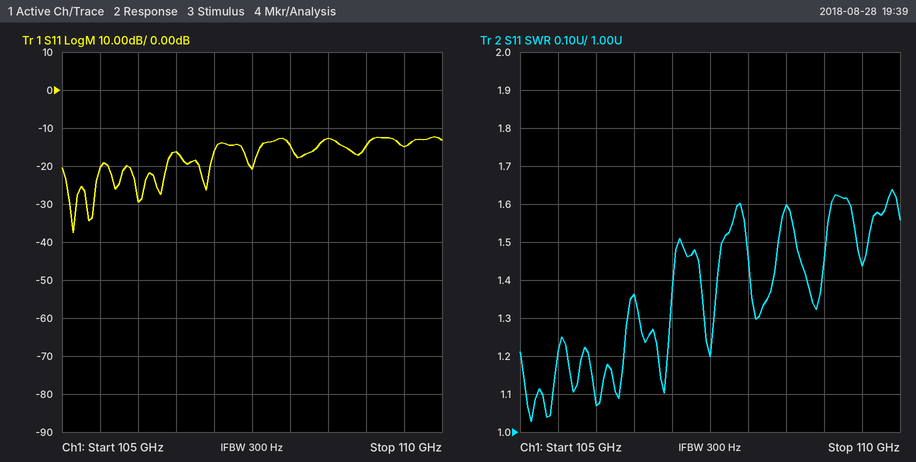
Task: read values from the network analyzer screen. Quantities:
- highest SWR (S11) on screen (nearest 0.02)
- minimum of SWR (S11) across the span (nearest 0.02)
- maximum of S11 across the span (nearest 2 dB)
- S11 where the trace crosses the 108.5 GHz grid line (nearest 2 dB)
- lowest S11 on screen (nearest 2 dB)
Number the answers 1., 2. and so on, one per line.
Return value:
1. 1.64
2. 1.02
3. -12 dB
4. -12 dB
5. -38 dB
